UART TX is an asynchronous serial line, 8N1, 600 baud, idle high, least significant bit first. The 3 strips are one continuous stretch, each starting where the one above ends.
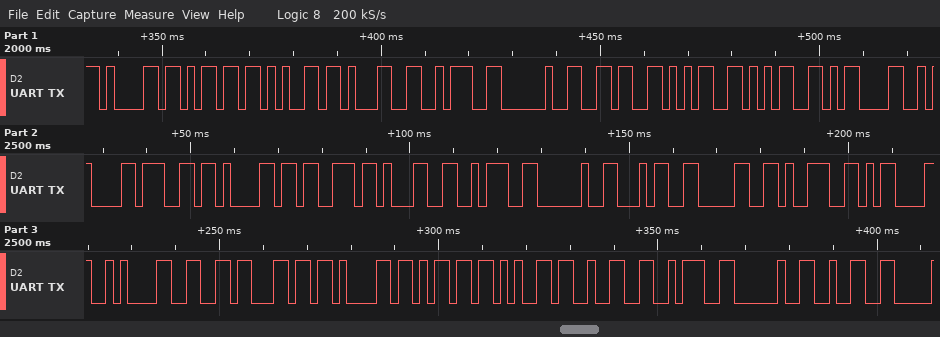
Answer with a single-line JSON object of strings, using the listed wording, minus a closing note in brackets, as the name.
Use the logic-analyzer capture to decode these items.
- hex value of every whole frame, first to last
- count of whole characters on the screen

{"hex value of every whole frame, first to last": "0x61 0x6D 0x65 0x31 0x3A 0x20 0x36 0x35 0x35 0x0D 0x0A 0x67 0x61 0x73 0x31 0x3A 0x20 0x34 0x30 0x39 0x0D 0x0A 0x66 0x6C 0x61 0x6D 0x65 0x32 0x3A 0x20 0x32", "count of whole characters on the screen": "31"}
